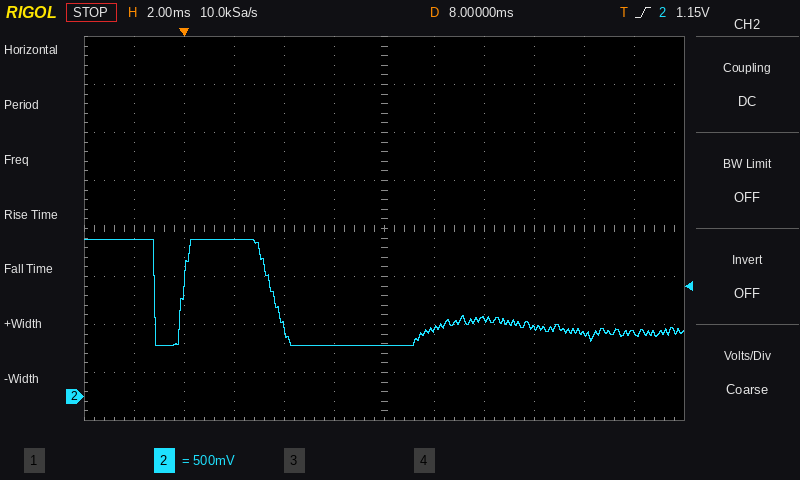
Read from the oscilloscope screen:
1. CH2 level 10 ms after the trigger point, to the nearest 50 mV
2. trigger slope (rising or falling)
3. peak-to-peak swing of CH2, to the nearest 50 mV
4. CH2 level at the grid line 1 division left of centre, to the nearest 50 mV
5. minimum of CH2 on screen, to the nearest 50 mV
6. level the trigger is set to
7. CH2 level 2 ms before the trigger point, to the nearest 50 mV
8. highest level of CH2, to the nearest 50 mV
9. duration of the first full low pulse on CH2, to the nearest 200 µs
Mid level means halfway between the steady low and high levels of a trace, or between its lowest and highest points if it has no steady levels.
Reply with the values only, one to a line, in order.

700 mV
rising
1.10 V
550 mV
550 mV
1.15 V
1.65 V
1.65 V
1.2 ms
